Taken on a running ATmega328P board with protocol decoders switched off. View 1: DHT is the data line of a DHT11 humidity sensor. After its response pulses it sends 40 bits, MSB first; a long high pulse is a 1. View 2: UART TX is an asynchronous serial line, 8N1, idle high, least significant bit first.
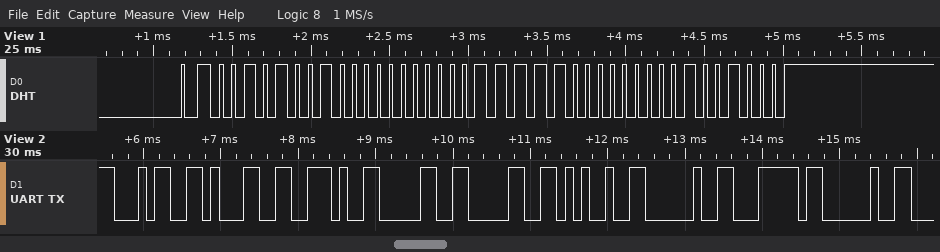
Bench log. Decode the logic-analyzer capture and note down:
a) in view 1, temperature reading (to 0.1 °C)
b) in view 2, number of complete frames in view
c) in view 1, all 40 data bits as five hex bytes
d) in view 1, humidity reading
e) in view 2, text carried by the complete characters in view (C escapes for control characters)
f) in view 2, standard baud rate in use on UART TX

31.0 °C
9
29 00 1F 00 48
41 %
"41.00% | "
9600 baud
